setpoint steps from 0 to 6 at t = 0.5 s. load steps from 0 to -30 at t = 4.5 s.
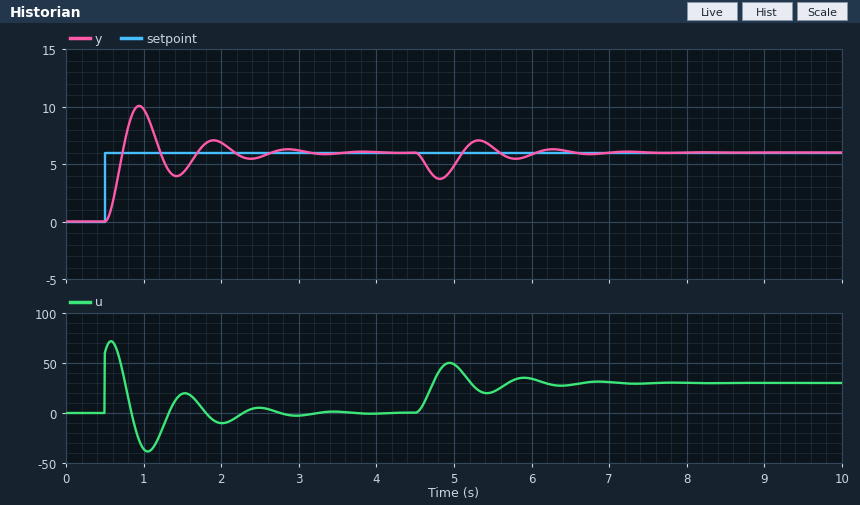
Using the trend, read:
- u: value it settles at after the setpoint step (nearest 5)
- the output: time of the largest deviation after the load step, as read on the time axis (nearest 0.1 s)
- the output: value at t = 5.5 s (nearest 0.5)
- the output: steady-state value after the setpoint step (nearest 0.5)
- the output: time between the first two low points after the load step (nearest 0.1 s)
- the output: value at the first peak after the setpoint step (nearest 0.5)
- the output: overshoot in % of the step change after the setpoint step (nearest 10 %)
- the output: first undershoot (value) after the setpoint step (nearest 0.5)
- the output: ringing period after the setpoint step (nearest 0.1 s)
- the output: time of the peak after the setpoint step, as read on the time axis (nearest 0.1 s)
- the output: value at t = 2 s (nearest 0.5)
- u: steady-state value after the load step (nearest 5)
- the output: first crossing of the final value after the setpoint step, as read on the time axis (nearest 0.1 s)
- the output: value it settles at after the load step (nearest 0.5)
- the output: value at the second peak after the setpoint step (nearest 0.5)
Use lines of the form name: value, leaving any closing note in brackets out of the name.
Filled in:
u: value it settles at after the setpoint step: 0
the output: time of the largest deviation after the load step, as read on the time axis: 4.8 s
the output: value at t = 5.5 s: 6.5
the output: steady-state value after the setpoint step: 6.0
the output: time between the first two low points after the load step: 1.0 s
the output: value at the first peak after the setpoint step: 10.0
the output: overshoot in % of the step change after the setpoint step: 70 %
the output: first undershoot (value) after the setpoint step: 4.0
the output: ringing period after the setpoint step: 1.0 s
the output: time of the peak after the setpoint step, as read on the time axis: 0.9 s
the output: value at t = 2 s: 7.0
u: steady-state value after the load step: 30
the output: first crossing of the final value after the setpoint step, as read on the time axis: 0.7 s
the output: value it settles at after the load step: 6.0
the output: value at the second peak after the setpoint step: 7.0
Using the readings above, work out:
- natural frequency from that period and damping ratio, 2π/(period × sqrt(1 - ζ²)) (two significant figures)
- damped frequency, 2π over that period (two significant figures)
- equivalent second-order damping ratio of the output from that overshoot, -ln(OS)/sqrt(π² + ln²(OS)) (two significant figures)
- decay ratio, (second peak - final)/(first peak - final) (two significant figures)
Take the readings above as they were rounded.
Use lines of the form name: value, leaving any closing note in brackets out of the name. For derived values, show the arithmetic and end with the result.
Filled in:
natural frequency from that period and damping ratio, 2π/(period × sqrt(1 - ζ²)): 2π / (1 × sqrt(1 - 0.11²)) = 6.3 rad/s
damped frequency, 2π over that period: 2π / 1 = 6.3 rad/s
equivalent second-order damping ratio of the output from that overshoot, -ln(OS)/sqrt(π² + ln²(OS)): ln(0.7) = -0.357; 0.357 / sqrt(9.870 + 0.127) = 0.11
decay ratio, (second peak - final)/(first peak - final): (7 - 6) / (10 - 6) = 0.25
